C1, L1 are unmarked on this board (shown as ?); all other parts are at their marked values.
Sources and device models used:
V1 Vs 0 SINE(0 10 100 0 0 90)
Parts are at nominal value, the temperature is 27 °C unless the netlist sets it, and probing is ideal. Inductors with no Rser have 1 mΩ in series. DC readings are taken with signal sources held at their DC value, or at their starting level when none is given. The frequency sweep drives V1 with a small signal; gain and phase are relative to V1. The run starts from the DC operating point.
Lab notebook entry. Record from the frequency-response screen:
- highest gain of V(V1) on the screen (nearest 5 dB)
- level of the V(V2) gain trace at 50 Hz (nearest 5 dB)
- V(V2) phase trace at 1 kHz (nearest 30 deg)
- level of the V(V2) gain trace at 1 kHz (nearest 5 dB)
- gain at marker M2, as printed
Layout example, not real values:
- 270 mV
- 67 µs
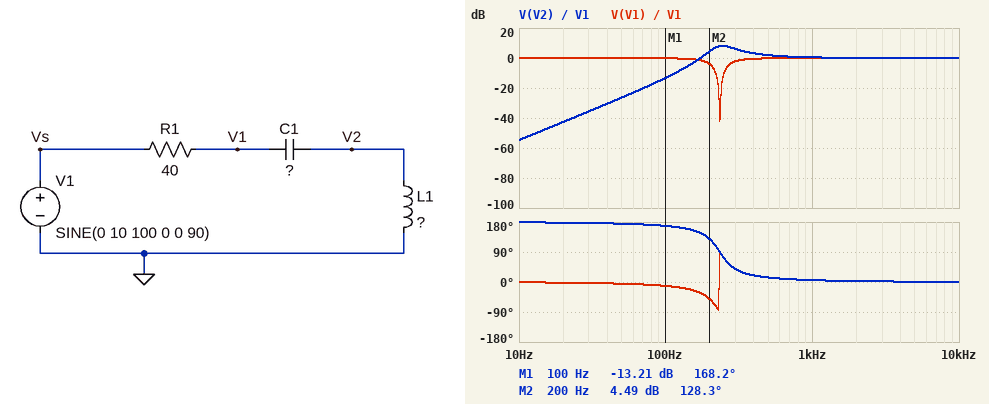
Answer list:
- 0 dB
- -25 dB
- 0 deg
- 0 dB
- 4.49 dB
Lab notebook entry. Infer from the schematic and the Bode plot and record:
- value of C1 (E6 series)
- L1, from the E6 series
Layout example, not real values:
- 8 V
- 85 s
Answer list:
- 6.8 µF
- 68 mH
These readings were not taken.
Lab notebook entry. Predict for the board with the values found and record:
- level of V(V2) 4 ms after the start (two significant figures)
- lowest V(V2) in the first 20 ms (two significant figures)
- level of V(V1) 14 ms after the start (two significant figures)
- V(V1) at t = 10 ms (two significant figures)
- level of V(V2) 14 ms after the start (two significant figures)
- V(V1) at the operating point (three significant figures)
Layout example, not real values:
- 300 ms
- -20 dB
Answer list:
- 1.9 V
- -2.2 V
- -6.6 V
- 9.5 V
- 1.5 V
- 10.0 V
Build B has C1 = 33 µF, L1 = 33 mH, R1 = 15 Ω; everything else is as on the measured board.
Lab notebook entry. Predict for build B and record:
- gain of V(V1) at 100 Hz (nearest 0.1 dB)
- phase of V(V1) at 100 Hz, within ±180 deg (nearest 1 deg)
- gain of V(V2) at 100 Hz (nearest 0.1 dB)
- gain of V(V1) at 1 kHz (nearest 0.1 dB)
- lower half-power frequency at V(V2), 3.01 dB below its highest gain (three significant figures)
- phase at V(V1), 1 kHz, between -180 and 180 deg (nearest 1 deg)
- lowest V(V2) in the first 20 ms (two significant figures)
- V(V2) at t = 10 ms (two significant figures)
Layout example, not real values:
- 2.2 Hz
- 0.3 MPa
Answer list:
- -1.1 dB
- -29 deg
- -3.6 dB
- 0 dB
- 131 Hz
- 4 deg
- -7.2 V
- -6.4 V
